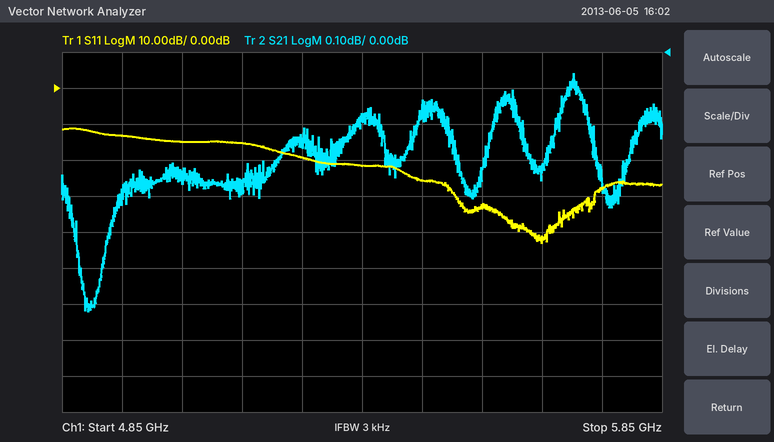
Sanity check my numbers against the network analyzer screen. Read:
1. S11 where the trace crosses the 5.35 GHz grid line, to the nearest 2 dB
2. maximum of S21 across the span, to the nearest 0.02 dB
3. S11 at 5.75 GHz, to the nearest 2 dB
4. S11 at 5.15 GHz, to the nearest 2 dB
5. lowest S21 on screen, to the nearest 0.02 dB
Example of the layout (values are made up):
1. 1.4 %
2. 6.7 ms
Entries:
1. -22 dB
2. -0.06 dB
3. -28 dB
4. -16 dB
5. -0.72 dB
